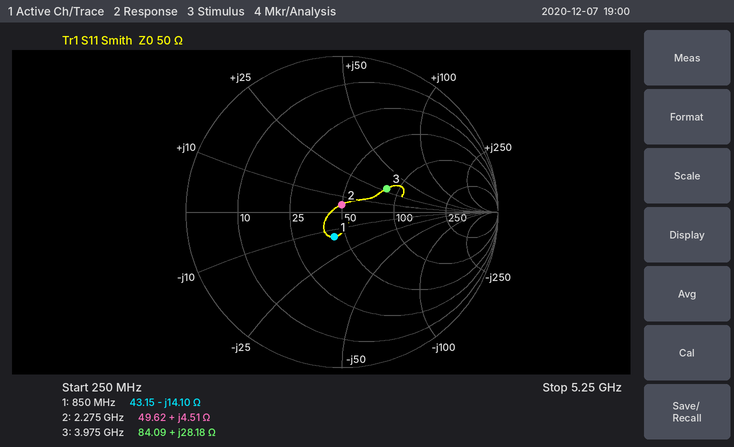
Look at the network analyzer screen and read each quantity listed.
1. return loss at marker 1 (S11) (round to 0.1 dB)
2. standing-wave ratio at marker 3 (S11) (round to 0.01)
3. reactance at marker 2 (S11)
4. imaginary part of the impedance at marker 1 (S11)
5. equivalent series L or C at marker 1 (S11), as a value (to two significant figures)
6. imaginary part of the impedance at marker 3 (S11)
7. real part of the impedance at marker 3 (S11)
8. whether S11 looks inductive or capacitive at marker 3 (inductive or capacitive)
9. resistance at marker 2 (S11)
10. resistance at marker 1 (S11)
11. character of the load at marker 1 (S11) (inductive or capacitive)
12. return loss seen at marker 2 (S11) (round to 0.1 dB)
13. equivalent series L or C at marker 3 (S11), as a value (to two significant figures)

15.6 dB
1.95
+4.51 Ω
-14.10 Ω
13 pF
+28.18 Ω
84.09 Ω
inductive
49.62 Ω
43.15 Ω
capacitive
26.9 dB
1.1 nH
